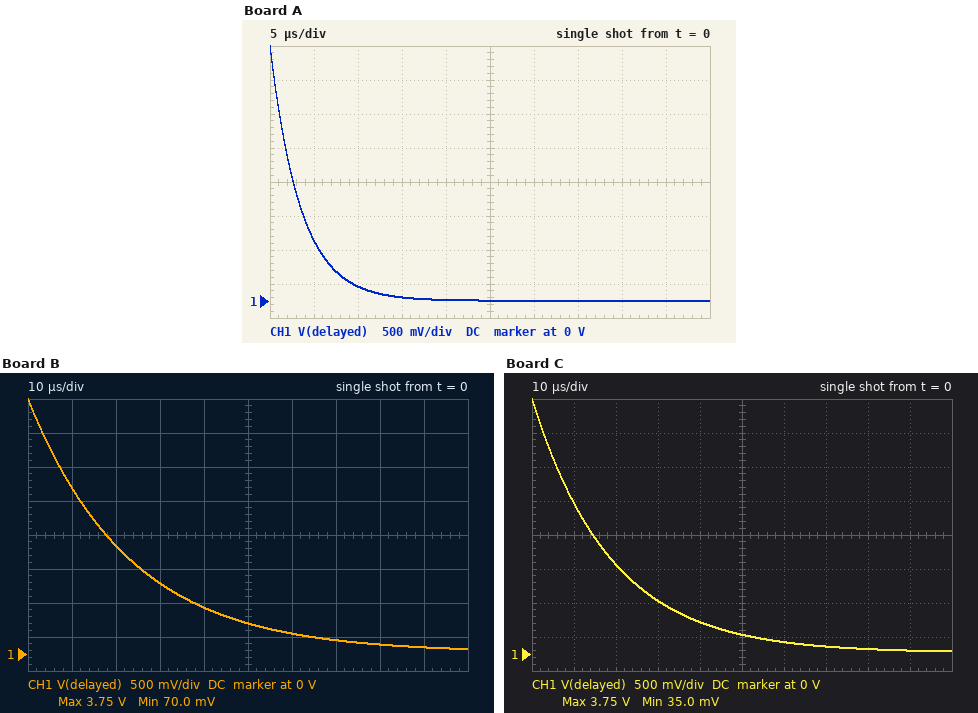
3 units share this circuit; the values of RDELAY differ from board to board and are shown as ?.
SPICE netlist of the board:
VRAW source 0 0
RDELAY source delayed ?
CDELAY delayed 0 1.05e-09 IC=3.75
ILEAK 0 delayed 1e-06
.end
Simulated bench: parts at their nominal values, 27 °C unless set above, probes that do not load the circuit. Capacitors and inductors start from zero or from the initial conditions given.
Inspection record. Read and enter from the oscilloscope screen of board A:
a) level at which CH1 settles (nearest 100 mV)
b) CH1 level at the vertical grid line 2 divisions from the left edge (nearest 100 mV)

0 V
200 mV
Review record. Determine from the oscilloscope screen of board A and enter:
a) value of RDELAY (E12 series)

3.3 kΩ
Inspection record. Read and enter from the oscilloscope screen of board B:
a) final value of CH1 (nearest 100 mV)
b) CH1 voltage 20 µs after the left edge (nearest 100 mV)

100 mV
1.6 V
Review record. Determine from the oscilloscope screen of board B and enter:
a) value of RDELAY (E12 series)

22 kΩ
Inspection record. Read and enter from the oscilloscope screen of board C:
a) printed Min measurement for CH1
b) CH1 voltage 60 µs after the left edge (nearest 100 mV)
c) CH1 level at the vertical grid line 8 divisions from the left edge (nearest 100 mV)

35.0 mV
200 mV
100 mV
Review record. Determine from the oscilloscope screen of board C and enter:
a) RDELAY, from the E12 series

18 kΩ
